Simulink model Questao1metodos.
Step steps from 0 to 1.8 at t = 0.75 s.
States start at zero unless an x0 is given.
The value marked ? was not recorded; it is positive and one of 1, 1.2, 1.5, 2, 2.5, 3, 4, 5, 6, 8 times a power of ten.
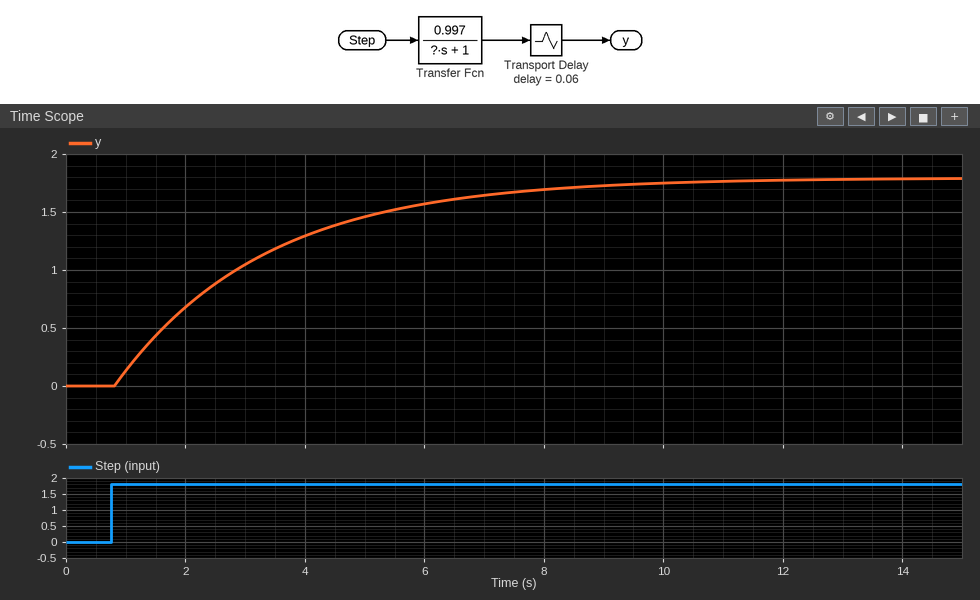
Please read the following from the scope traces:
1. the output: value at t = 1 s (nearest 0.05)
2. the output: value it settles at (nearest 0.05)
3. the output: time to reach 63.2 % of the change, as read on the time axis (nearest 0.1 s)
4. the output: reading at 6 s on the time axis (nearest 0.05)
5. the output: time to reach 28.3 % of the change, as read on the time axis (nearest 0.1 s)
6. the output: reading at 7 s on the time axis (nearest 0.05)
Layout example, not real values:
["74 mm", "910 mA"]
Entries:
["0.15", "1.80", "3.3 s", "1.55", "1.6 s", "1.65"]
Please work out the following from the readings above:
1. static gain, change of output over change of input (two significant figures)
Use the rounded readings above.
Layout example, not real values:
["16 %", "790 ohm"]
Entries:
["1.0"]
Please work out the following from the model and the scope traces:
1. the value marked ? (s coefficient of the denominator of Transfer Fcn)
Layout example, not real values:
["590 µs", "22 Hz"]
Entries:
["2.5"]
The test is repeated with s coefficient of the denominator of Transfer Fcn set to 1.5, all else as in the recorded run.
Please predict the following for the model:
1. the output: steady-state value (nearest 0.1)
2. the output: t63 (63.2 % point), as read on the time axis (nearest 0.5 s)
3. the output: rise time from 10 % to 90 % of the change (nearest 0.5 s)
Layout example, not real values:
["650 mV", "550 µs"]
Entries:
["1.8", "2.5 s", "3.5 s"]
